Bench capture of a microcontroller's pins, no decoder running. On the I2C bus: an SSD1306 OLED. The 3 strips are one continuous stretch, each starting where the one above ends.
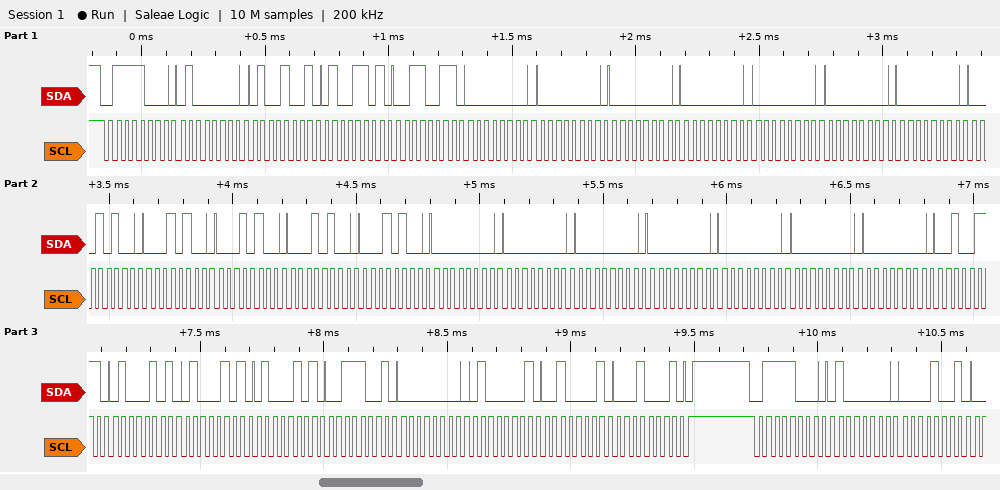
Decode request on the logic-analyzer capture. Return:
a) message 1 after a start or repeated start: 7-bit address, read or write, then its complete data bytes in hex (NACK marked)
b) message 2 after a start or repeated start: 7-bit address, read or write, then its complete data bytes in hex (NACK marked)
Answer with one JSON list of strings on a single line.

["0x3C write: 40 49 4D 33 00 00 00 00 00 00 00 14 14 14 14 14 00 00 00 00 00 00 00 27 45 45 45 39 00 41 21 11", "0x3C write: 40 09"]
